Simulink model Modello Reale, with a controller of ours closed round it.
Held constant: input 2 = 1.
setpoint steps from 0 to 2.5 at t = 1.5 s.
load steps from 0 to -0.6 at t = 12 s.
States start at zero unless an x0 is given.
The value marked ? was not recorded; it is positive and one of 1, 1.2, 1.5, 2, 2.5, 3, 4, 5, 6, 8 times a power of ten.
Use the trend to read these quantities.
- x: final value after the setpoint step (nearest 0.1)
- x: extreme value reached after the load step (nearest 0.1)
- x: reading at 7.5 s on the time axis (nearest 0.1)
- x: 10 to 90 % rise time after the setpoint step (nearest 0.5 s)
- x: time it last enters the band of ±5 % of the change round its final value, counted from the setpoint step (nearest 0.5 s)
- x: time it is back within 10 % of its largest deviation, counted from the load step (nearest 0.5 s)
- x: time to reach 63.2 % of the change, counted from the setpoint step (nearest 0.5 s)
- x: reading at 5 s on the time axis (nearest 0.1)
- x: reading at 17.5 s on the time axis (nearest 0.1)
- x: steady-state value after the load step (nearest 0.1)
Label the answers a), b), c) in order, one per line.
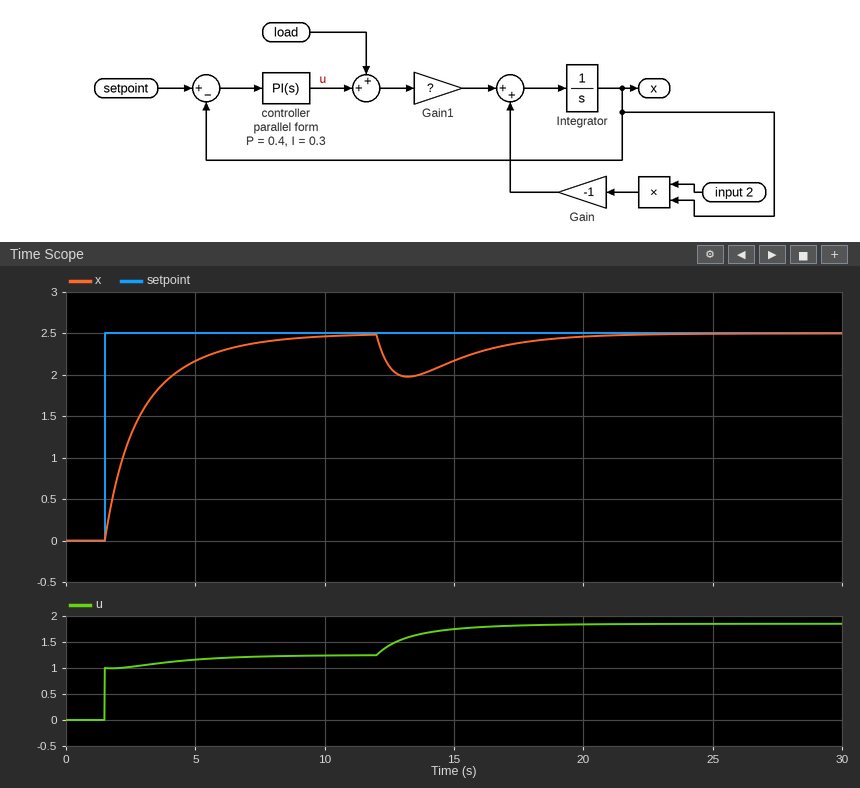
a) 2.5
b) 2.0
c) 2.4
d) 4.0 s
e) 5.5 s
f) 7.5 s
g) 1.5 s
h) 2.2
i) 2.4
j) 2.5
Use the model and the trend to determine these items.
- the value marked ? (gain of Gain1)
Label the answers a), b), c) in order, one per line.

a) 2
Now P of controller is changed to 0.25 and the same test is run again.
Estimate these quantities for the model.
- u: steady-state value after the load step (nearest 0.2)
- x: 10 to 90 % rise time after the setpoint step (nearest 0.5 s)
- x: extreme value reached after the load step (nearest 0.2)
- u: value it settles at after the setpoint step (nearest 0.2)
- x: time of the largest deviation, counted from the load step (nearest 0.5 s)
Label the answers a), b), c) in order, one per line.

a) 1.8
b) 3.5 s
c) 2.0
d) 1.2
e) 1.5 s
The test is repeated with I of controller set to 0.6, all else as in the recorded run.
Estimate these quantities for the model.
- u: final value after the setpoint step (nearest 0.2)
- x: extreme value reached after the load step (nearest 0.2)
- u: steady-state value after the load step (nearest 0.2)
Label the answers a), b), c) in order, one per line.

a) 1.2
b) 2.0
c) 1.8
